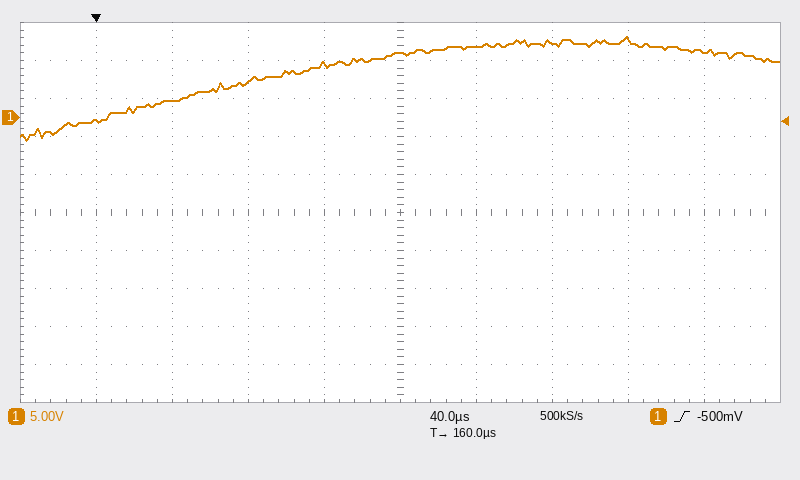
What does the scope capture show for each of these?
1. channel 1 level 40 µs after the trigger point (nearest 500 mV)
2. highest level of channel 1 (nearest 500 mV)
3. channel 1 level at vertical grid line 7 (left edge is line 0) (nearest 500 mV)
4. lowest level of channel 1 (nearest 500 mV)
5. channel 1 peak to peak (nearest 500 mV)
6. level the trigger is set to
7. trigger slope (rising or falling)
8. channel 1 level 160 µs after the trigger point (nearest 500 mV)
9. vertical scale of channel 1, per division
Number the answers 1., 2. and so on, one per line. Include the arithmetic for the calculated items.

1. 2.0 V
2. 10.5 V
3. 10.0 V
4. -3.0 V
5. 10.5 V − (-3.0 V) = 13.5 V
6. -500 mV
7. rising
8. 8.5 V
9. 5 V
